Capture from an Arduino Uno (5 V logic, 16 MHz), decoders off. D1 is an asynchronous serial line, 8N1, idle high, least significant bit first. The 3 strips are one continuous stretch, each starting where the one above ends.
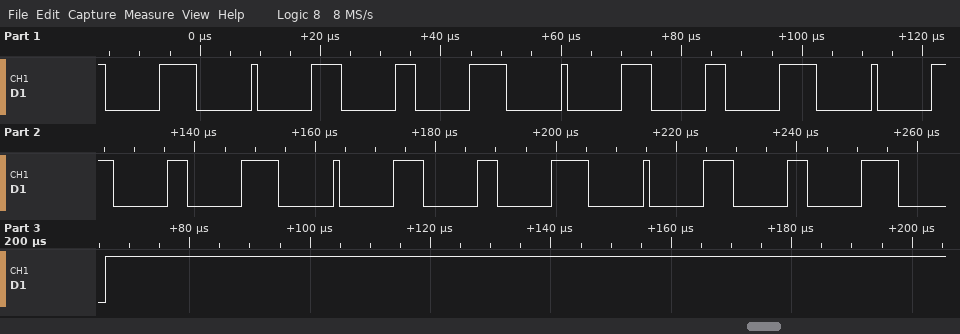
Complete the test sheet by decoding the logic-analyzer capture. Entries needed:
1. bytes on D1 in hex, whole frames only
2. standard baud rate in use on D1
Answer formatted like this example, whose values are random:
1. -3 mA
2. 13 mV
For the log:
1. 0x00 0x00 0x00 0x00 0x00 0x00 0x00 0x00 0x00 0x00 0x00 0x00 0x00 0x00 0x00 0x00 0x00 0x00 0x00 0x00 0x00 0x00
2. 1000000 baud
